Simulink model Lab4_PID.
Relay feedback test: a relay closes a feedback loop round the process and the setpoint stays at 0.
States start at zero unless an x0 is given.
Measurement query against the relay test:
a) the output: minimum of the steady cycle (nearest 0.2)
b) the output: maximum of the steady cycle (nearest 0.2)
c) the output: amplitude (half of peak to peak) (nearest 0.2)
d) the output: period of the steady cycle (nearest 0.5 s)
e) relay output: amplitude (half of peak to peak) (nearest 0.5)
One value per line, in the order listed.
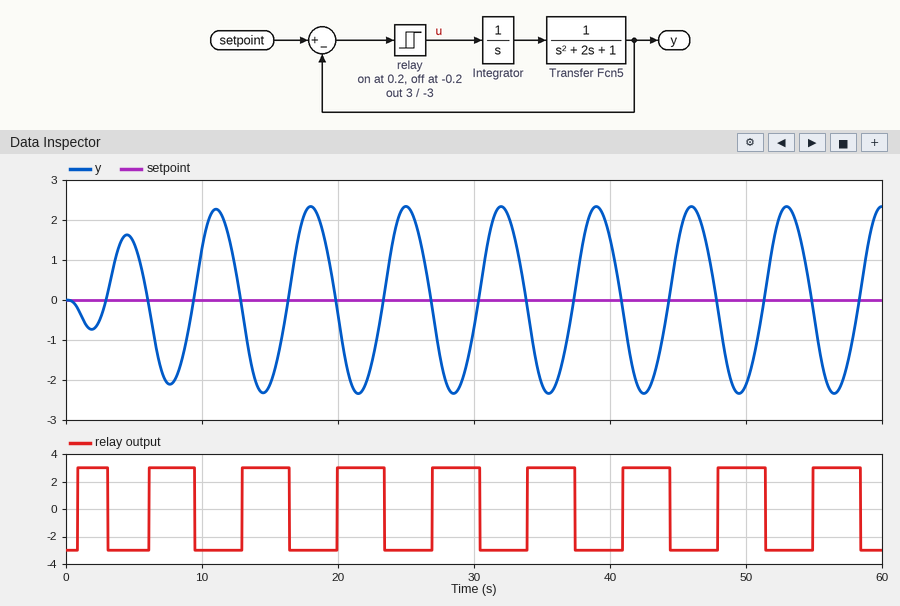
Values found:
-2.4
2.4
2.4
7.0 s
3.0
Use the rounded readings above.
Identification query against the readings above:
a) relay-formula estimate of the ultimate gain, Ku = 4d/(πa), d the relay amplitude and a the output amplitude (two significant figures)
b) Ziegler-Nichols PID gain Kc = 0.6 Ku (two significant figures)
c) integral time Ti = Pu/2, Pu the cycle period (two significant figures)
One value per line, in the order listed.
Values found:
1.6
0.96
3.5 s
